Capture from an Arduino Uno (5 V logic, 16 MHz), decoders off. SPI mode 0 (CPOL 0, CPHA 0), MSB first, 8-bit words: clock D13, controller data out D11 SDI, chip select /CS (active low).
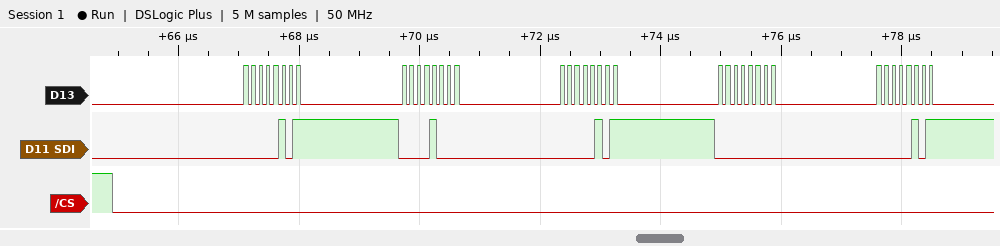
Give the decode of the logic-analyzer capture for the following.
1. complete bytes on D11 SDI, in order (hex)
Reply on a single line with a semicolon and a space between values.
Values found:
05 08 05 00 05
